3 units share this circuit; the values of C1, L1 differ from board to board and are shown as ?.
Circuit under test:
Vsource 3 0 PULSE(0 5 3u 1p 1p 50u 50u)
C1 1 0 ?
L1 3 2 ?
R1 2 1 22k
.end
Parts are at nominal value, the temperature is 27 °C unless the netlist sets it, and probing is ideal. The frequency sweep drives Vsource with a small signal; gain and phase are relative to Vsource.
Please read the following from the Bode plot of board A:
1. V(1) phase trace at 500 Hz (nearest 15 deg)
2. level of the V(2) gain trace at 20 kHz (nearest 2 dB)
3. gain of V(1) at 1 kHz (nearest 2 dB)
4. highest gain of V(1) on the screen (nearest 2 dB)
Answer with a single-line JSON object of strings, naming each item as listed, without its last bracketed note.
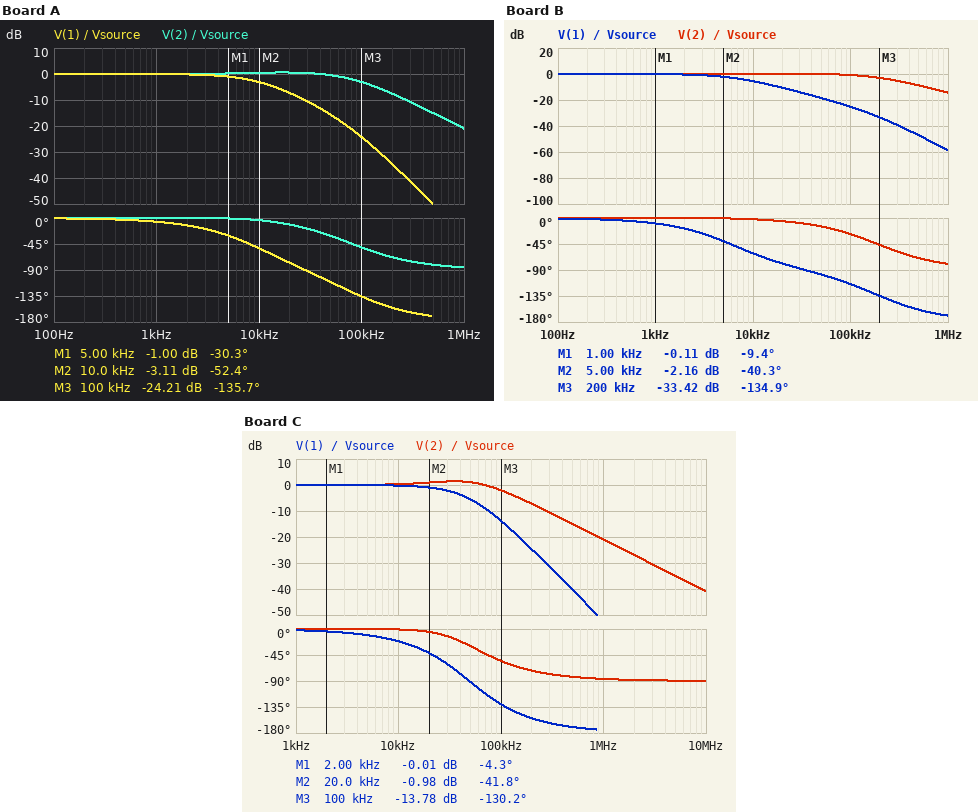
{"V(1) phase trace at 500 Hz": "0 deg", "level of the V(2) gain trace at 20 kHz": "0 dB", "gain of V(1) at 1 kHz": "0 dB", "highest gain of V(1) on the screen": "0 dB"}
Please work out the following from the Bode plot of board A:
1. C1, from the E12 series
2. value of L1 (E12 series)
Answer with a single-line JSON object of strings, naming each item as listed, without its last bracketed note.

{"C1, from the E12 series": "820 pF", "value of L1": "39 mH"}
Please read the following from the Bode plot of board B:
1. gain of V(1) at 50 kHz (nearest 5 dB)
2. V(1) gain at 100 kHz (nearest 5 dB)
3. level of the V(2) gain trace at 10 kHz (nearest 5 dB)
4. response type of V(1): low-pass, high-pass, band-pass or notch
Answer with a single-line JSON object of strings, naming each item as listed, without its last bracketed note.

{"gain of V(1) at 50 kHz": "-20 dB", "V(1) gain at 100 kHz": "-25 dB", "level of the V(2) gain trace at 10 kHz": "0 dB", "response type of V(1): low-pass, high-pass, band-pass or notch": "low-pass"}
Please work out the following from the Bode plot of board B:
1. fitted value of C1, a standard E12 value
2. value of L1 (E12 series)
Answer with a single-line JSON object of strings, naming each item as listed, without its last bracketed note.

{"fitted value of C1, a standard E12 value": "1.2 nF", "value of L1": "18 mH"}
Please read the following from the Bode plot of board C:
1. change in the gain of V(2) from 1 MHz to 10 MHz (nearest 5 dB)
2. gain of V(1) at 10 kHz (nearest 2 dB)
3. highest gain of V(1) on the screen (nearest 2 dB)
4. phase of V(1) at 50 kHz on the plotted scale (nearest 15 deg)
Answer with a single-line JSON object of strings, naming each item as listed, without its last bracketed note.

{"change in the gain of V(2) from 1 MHz to 10 MHz": "-20 dB", "gain of V(1) at 10 kHz": "0 dB", "highest gain of V(1) on the screen": "0 dB", "phase of V(1) at 50 kHz on the plotted scale": "-90 deg"}
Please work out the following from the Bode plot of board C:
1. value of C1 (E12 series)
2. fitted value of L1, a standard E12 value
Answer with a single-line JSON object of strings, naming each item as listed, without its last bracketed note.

{"value of C1": "270 pF", "fitted value of L1, a standard E12 value": "39 mH"}
